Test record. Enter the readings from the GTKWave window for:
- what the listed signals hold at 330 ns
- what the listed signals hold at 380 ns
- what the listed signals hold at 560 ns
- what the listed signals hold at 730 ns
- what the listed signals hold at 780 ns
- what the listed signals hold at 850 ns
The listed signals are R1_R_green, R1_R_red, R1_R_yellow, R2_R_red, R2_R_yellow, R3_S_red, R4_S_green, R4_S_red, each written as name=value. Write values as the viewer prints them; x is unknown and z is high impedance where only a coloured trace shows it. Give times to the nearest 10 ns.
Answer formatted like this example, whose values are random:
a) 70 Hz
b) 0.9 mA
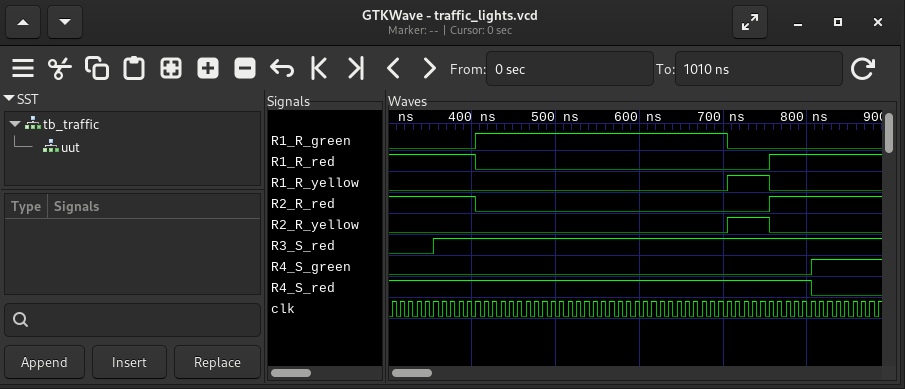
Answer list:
a) R1_R_green=0, R1_R_red=1, R1_R_yellow=0, R2_R_red=1, R2_R_yellow=0, R3_S_red=0, R4_S_green=0, R4_S_red=1
b) R1_R_green=0, R1_R_red=1, R1_R_yellow=0, R2_R_red=1, R2_R_yellow=0, R3_S_red=1, R4_S_green=0, R4_S_red=1
c) R1_R_green=1, R1_R_red=0, R1_R_yellow=0, R2_R_red=0, R2_R_yellow=0, R3_S_red=1, R4_S_green=0, R4_S_red=1
d) R1_R_green=0, R1_R_red=0, R1_R_yellow=1, R2_R_red=0, R2_R_yellow=1, R3_S_red=1, R4_S_green=0, R4_S_red=1
e) R1_R_green=0, R1_R_red=1, R1_R_yellow=0, R2_R_red=1, R2_R_yellow=0, R3_S_red=1, R4_S_green=0, R4_S_red=1
f) R1_R_green=0, R1_R_red=1, R1_R_yellow=0, R2_R_red=1, R2_R_yellow=0, R3_S_red=1, R4_S_green=1, R4_S_red=0
